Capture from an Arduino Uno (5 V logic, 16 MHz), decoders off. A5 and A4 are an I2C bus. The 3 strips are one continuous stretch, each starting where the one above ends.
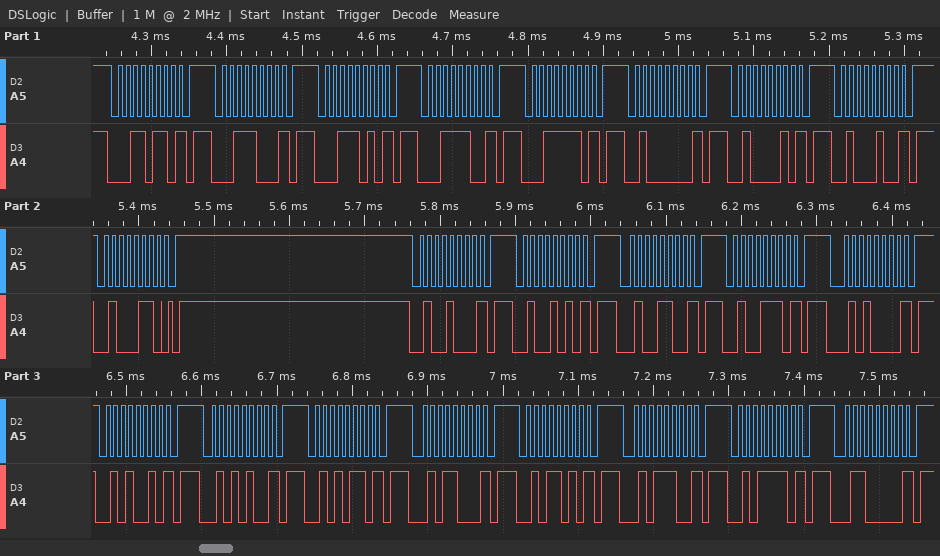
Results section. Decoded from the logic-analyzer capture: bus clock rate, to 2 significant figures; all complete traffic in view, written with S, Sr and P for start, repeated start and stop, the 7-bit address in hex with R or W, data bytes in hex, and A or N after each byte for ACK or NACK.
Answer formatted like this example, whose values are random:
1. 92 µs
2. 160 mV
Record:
1. 100 kHz
2. S 1BW N P S 1CW N P S 1DW N P S 1EW N P S 1FW N P S 20W N P S 21W N P S 22W N P S 23W A P S 24W N P S 25W N P S 26W N P S 27W N P S 28W N P S 29W N P S 2AW N P S 2BW N P S 2CW N P S 2DW N P S 2EW N P S 2FW N P S 30W N P
